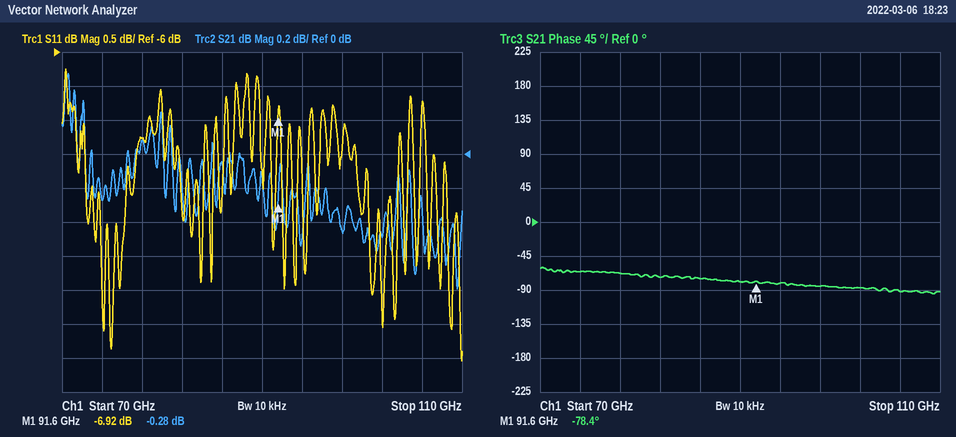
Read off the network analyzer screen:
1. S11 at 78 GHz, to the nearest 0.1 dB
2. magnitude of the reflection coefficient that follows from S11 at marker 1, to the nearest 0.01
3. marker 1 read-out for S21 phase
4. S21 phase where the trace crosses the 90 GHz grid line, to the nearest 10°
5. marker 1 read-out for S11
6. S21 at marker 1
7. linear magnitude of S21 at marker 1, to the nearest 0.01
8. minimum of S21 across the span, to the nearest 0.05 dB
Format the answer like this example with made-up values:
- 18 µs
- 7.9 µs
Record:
- -7.3 dB
- 0.45
- -78.4°
- -80°
- -6.92 dB
- -0.28 dB
- 0.97
- -0.80 dB
